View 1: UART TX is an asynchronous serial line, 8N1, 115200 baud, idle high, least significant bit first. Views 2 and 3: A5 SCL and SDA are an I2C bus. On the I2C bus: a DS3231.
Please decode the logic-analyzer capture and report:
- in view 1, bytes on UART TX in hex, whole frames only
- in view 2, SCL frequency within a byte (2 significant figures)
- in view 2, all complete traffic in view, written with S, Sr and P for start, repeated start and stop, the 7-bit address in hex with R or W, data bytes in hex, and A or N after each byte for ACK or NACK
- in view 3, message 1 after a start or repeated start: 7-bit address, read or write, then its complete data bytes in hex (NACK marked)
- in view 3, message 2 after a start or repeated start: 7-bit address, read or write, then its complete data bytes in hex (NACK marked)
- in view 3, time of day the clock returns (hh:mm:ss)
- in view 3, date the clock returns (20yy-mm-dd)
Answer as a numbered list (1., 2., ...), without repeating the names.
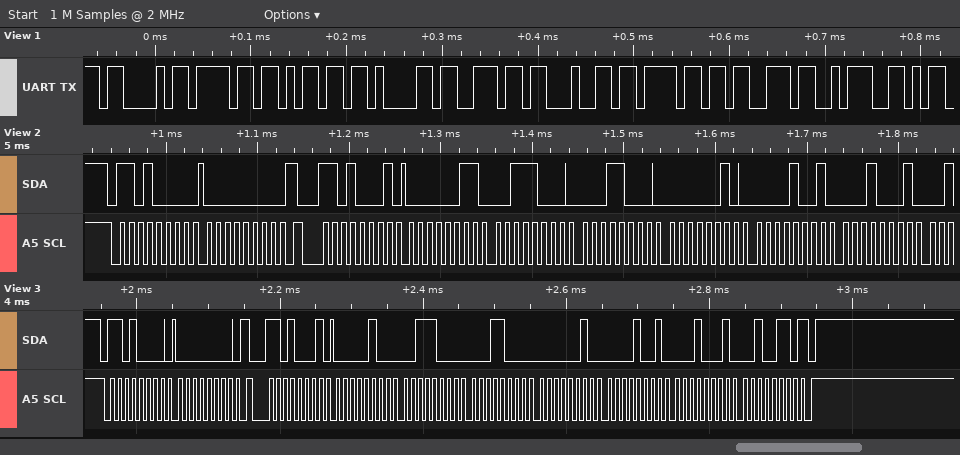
1. 0x43 0x6F 0x6D 0x61 0x6E 0x64 0x6F 0x73 0x3A
2. 100 kHz
3. S 68W A 00 A Sr 68R A 03 A 38 A 18 A 02 A 09 A 11 A
4. 0x68 write: 00
5. 0x68 read: 04 38 18 02 09 11 26 NACK
6. 18:38:04
7. 2026-11-09
